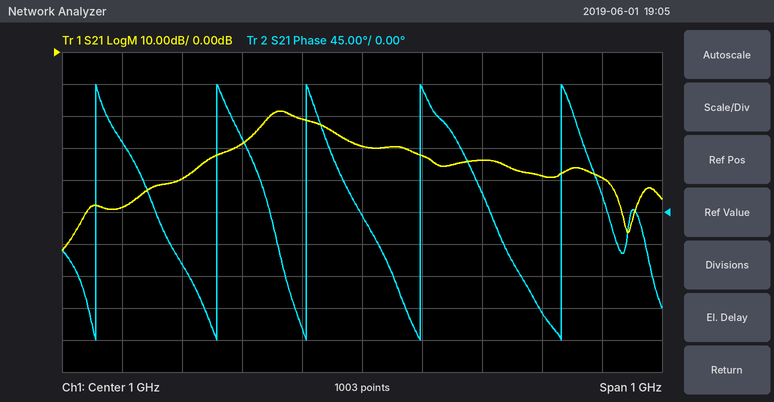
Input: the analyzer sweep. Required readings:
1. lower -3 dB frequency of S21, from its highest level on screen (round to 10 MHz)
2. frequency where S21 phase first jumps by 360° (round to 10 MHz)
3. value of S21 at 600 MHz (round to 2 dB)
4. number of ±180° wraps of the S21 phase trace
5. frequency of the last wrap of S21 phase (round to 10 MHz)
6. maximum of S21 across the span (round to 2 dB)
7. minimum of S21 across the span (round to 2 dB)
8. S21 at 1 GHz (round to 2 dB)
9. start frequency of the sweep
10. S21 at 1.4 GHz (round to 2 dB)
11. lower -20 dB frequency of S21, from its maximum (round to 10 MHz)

840 MHz
560 MHz
-48 dB
5
1.33 GHz
-18 dB
-62 dB
-30 dB
500 MHz
-40 dB
710 MHz
